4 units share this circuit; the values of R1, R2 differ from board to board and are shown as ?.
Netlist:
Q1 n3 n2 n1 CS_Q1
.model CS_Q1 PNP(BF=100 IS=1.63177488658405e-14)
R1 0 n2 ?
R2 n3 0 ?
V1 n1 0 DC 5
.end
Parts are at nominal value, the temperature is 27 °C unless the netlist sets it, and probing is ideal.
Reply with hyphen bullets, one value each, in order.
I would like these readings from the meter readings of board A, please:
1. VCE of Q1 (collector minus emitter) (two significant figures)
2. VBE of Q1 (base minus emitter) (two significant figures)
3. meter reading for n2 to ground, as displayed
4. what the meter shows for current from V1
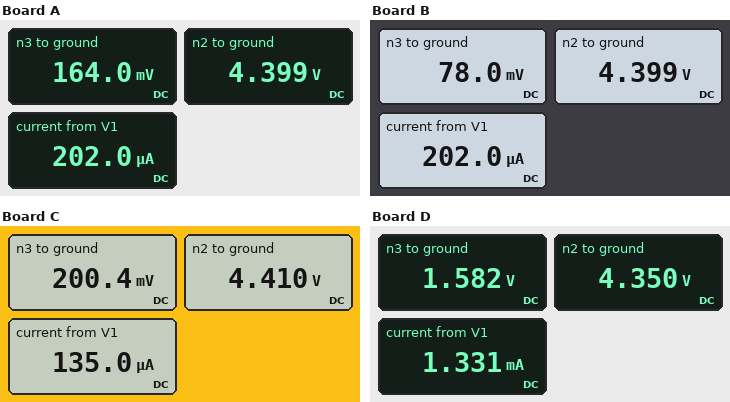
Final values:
- -4.8 V
- -600 mV
- 4.399 V
- 202.0 µA
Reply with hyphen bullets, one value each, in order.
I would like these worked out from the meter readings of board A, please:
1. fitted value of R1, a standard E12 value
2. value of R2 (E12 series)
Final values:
- 2.2 MΩ
- 820 Ω
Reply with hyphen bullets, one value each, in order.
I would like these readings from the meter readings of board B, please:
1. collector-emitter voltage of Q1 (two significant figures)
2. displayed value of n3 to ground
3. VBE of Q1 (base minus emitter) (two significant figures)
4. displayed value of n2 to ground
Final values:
- -4.9 V
- 78.0 mV
- -600 mV
- 4.399 V
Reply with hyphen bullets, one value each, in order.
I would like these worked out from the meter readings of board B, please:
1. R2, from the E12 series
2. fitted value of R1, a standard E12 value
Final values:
- 390 Ω
- 2.2 MΩ
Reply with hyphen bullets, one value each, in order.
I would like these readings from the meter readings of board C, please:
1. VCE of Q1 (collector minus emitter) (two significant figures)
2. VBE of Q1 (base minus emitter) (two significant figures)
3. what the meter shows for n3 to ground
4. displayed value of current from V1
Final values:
- -4.8 V
- -590 mV
- 200.4 mV
- 135.0 µA
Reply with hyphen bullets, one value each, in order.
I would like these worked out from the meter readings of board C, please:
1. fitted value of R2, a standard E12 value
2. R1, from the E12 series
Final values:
- 1.5 kΩ
- 3.3 MΩ
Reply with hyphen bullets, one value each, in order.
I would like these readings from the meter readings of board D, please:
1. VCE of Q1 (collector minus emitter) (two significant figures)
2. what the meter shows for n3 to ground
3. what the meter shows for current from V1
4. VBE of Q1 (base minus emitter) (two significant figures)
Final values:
- -3.4 V
- 1.582 V
- 1.331 mA
- -650 mV
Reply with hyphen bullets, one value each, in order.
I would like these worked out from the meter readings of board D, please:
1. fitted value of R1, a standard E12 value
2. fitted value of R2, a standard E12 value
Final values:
- 330 kΩ
- 1.2 kΩ
